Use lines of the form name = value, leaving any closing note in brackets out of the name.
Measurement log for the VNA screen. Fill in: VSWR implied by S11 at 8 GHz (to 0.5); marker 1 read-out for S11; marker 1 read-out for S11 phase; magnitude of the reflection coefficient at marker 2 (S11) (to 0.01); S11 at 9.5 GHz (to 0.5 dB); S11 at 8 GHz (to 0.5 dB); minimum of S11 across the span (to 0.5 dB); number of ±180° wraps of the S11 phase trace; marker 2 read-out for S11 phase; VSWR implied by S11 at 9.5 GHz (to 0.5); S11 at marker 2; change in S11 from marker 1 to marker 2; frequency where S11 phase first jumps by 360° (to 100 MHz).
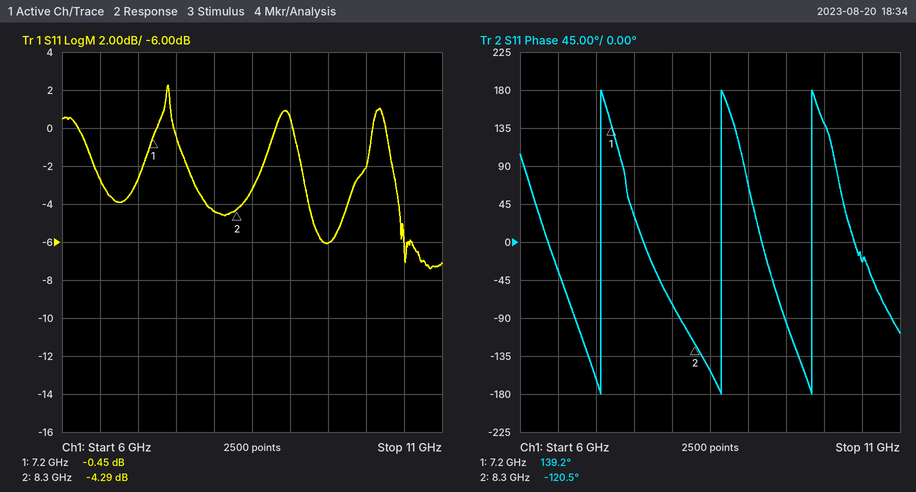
VSWR implied by S11 at 8 GHz = 4.0
marker 1 read-out for S11 = -0.45 dB
marker 1 read-out for S11 phase = 139.2°
magnitude of the reflection coefficient at marker 2 (S11) = 0.61
S11 at 9.5 GHz = -6.0 dB
S11 at 8 GHz = -4.5 dB
minimum of S11 across the span = -7.5 dB
number of ±180° wraps of the S11 phase trace = 3
marker 2 read-out for S11 phase = -120.5°
VSWR implied by S11 at 9.5 GHz = 3.0
S11 at marker 2 = -4.29 dB
change in S11 from marker 1 to marker 2 = -3.84 dB
frequency where S11 phase first jumps by 360° = 7.1 GHz
